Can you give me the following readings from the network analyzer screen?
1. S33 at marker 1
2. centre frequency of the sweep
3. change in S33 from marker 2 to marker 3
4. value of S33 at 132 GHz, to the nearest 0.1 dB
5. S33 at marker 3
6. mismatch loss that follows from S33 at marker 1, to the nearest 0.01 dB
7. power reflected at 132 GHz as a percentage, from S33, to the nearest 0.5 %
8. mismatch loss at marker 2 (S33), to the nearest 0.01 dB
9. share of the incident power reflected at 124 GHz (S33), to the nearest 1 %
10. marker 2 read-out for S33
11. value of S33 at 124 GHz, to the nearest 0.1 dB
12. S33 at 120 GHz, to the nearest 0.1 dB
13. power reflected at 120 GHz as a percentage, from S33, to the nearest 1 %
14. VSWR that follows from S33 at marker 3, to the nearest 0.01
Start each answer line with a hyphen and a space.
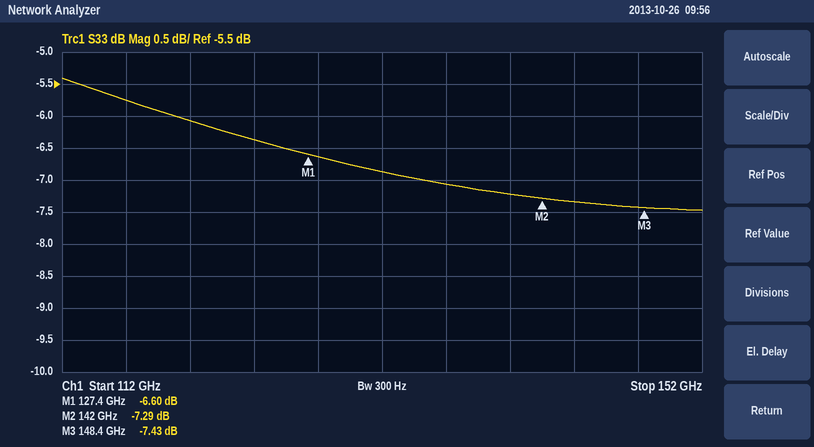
- -6.60 dB
- 132 GHz
- -0.14 dB
- -6.9 dB
- -7.43 dB
- 1.07 dB
- 20.5 %
- 0.90 dB
- 23 %
- -7.29 dB
- -6.4 dB
- -6.1 dB
- 25 %
- 2.48
